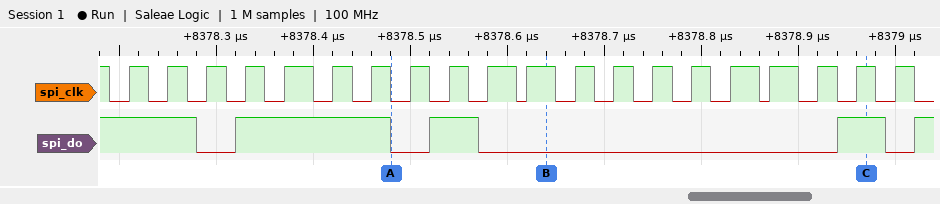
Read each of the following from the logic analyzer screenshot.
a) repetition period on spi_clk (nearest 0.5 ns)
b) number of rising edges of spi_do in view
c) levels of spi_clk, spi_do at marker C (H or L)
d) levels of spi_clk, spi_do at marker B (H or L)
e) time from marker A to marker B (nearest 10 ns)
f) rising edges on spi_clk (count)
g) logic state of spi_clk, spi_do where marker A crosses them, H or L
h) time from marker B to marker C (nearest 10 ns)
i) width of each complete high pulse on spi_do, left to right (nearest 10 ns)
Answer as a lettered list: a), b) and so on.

a) 41.5 ns
b) 4
c) spi_clk=H, spi_do=H
d) spi_clk=H, spi_do=L
e) 160 ns
f) 20
g) spi_clk=L, spi_do=L
h) 330 ns
i) 160 ns, 50 ns, 50 ns
